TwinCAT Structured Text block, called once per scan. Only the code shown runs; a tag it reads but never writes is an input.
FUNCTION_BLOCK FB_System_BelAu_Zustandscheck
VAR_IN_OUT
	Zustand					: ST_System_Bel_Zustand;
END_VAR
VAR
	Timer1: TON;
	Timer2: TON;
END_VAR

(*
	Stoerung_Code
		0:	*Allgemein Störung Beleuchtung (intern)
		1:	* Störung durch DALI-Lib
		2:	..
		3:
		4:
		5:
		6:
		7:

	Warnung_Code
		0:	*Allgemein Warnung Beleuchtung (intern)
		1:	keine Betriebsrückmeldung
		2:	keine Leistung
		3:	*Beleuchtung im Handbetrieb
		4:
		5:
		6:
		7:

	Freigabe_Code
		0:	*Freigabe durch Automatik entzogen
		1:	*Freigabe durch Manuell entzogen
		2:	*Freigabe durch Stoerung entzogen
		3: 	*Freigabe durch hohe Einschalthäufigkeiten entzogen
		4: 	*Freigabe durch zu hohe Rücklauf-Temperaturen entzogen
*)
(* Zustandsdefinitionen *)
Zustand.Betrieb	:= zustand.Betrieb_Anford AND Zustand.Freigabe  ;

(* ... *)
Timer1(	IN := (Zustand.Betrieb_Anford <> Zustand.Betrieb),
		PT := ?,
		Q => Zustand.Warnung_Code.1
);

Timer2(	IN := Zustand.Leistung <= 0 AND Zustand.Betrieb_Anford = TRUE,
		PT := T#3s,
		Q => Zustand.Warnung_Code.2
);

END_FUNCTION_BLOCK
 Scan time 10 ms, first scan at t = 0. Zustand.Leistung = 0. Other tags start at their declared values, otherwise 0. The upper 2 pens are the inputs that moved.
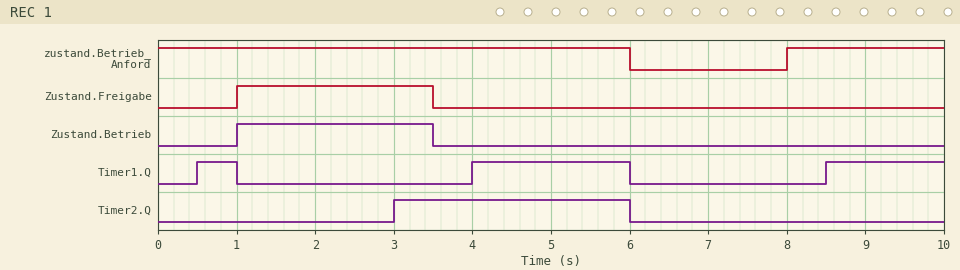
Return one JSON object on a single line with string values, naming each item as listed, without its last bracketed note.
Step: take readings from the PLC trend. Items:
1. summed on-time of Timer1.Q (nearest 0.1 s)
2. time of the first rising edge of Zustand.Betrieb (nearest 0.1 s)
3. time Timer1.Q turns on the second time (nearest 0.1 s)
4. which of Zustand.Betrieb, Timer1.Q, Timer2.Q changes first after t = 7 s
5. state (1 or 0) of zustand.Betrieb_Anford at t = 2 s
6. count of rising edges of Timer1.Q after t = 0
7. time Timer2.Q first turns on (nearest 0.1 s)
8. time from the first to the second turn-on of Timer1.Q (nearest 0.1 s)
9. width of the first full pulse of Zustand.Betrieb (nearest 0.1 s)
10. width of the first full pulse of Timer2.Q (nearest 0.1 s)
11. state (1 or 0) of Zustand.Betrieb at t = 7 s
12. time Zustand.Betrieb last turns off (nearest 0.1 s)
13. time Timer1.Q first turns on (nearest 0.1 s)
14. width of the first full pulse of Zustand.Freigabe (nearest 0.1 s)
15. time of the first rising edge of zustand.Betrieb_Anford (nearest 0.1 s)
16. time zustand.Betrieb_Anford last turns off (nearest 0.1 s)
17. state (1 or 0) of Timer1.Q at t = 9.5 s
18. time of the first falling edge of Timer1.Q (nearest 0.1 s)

{"summed on-time of Timer1.Q": "4.0 s", "time of the first rising edge of Zustand.Betrieb": "1.0 s", "time Timer1.Q turns on the second time": "4.0 s", "which of Zustand.Betrieb, Timer1.Q, Timer2.Q changes first after t = 7 s": "Timer1.Q", "state (1 or 0) of zustand.Betrieb_Anford at t = 2 s": "1", "count of rising edges of Timer1.Q after t = 0": "3", "time Timer2.Q first turns on": "3.0 s", "time from the first to the second turn-on of Timer1.Q": "3.5 s", "width of the first full pulse of Zustand.Betrieb": "2.5 s", "width of the first full pulse of Timer2.Q": "3.0 s", "state (1 or 0) of Zustand.Betrieb at t = 7 s": "0", "time Zustand.Betrieb last turns off": "3.5 s", "time Timer1.Q first turns on": "0.5 s", "width of the first full pulse of Zustand.Freigabe": "2.5 s", "time of the first rising edge of zustand.Betrieb_Anford": "8.0 s", "time zustand.Betrieb_Anford last turns off": "6.0 s", "state (1 or 0) of Timer1.Q at t = 9.5 s": "1", "time of the first falling edge of Timer1.Q": "1.0 s"}
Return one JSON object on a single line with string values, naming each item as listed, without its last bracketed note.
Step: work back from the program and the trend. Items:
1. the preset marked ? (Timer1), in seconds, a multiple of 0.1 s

{"the preset marked ? (Timer1), in seconds, a multiple of 0.1 s": "0.5 s"}
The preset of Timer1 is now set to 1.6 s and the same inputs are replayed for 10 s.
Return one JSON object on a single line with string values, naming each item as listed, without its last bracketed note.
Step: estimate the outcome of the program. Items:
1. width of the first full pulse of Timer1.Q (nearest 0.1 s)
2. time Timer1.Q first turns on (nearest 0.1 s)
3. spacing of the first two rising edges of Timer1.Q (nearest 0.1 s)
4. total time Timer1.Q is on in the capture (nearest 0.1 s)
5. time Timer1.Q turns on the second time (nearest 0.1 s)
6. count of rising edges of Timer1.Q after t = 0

{"width of the first full pulse of Timer1.Q": "0.9 s", "time Timer1.Q first turns on": "5.1 s", "spacing of the first two rising edges of Timer1.Q": "4.5 s", "total time Timer1.Q is on in the capture": "1.3 s", "time Timer1.Q turns on the second time": "9.6 s", "count of rising edges of Timer1.Q after t = 0": "2"}
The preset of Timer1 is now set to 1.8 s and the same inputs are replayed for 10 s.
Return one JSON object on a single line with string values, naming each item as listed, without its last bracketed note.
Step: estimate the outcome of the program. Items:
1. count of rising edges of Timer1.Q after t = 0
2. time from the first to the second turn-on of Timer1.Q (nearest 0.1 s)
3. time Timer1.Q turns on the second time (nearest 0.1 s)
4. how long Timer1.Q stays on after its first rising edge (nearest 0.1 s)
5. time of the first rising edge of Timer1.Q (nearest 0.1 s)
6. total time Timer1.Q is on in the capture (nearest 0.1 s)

{"count of rising edges of Timer1.Q after t = 0": "2", "time from the first to the second turn-on of Timer1.Q": "4.5 s", "time Timer1.Q turns on the second time": "9.8 s", "how long Timer1.Q stays on after its first rising edge": "0.7 s", "time of the first rising edge of Timer1.Q": "5.3 s", "total time Timer1.Q is on in the capture": "0.9 s"}
